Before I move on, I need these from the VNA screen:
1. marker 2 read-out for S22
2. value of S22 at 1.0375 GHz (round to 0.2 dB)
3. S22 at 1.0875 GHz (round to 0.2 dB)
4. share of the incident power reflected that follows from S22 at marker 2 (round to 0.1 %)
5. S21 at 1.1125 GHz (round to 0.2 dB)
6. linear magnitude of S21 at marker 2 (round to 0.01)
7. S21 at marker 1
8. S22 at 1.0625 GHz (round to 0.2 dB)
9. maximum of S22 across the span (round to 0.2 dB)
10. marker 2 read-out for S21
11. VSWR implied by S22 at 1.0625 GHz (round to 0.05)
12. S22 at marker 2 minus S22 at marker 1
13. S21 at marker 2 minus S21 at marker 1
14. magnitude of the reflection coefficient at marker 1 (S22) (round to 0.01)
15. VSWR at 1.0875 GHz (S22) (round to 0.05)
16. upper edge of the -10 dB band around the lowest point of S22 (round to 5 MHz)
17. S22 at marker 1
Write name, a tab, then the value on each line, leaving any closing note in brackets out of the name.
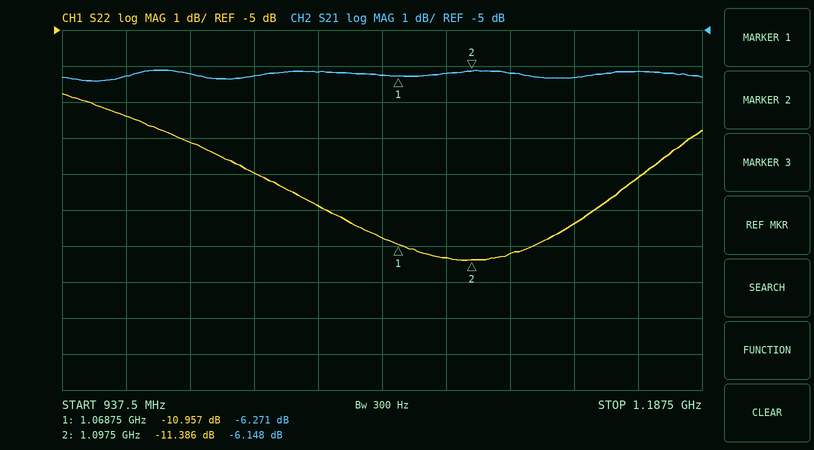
marker 2 read-out for S22	-11.386 dB
value of S22 at 1.0375 GHz	-9.8 dB
S22 at 1.0875 GHz	-11.4 dB
share of the incident power reflected that follows from S22 at marker 2	7.3 %
S21 at 1.1125 GHz	-6.2 dB
linear magnitude of S21 at marker 2	0.49
S21 at marker 1	-6.271 dB
S22 at 1.0625 GHz	-10.8 dB
maximum of S22 across the span	-6.8 dB
marker 2 read-out for S21	-6.148 dB
VSWR implied by S22 at 1.0625 GHz	1.80
S22 at marker 2 minus S22 at marker 1	-0.429 dB
S21 at marker 2 minus S21 at marker 1	0.123 dB
magnitude of the reflection coefficient at marker 1 (S22)	0.28
VSWR at 1.0875 GHz (S22)	1.75
upper edge of the -10 dB band around the lowest point of S22	1.145 GHz
S22 at marker 1	-10.957 dB
